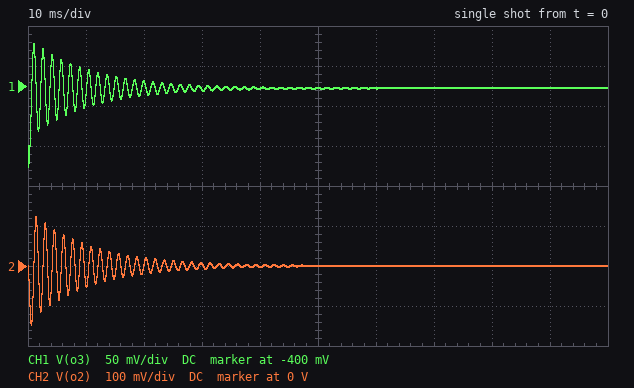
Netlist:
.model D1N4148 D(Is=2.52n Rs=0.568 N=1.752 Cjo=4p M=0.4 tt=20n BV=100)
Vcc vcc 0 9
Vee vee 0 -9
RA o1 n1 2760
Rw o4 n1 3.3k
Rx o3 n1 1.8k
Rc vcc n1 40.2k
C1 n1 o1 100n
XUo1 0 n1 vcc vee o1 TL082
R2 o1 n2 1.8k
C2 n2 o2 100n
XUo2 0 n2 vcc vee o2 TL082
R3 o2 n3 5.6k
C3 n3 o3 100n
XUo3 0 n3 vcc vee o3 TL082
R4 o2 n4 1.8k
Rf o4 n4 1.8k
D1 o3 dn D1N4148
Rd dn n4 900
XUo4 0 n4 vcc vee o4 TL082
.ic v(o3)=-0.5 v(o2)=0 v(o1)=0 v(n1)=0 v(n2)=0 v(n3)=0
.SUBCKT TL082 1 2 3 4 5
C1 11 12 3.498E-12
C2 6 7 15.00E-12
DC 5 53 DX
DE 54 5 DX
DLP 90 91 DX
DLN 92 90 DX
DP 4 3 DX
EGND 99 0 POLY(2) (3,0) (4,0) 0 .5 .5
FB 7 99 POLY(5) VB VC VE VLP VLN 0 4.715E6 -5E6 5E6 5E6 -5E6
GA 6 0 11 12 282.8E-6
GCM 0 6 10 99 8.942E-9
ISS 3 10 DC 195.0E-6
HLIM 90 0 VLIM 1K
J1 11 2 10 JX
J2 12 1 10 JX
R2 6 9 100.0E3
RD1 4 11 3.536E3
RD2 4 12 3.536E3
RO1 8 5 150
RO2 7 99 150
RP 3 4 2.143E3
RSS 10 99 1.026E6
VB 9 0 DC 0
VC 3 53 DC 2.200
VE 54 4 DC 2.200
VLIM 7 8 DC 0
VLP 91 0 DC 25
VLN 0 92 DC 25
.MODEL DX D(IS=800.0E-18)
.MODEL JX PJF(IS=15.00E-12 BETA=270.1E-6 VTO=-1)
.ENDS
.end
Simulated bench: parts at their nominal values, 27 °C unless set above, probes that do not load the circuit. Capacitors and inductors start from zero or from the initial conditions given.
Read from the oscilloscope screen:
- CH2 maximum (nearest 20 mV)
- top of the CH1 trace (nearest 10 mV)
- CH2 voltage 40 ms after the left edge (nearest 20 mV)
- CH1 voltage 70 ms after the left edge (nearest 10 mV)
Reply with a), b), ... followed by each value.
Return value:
a) 120 mV
b) -350 mV
c) 0 V
d) -400 mV
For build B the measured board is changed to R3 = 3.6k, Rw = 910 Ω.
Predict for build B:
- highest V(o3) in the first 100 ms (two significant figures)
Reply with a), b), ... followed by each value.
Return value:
a) -400 mV
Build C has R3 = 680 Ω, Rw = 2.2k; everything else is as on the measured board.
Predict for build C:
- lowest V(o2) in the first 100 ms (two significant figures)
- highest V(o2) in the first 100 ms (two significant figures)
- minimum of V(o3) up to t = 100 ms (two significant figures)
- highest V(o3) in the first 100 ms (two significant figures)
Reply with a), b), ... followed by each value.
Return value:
a) -6.8 V
b) 3.1 V
c) -7.3 V
d) 7.5 V
